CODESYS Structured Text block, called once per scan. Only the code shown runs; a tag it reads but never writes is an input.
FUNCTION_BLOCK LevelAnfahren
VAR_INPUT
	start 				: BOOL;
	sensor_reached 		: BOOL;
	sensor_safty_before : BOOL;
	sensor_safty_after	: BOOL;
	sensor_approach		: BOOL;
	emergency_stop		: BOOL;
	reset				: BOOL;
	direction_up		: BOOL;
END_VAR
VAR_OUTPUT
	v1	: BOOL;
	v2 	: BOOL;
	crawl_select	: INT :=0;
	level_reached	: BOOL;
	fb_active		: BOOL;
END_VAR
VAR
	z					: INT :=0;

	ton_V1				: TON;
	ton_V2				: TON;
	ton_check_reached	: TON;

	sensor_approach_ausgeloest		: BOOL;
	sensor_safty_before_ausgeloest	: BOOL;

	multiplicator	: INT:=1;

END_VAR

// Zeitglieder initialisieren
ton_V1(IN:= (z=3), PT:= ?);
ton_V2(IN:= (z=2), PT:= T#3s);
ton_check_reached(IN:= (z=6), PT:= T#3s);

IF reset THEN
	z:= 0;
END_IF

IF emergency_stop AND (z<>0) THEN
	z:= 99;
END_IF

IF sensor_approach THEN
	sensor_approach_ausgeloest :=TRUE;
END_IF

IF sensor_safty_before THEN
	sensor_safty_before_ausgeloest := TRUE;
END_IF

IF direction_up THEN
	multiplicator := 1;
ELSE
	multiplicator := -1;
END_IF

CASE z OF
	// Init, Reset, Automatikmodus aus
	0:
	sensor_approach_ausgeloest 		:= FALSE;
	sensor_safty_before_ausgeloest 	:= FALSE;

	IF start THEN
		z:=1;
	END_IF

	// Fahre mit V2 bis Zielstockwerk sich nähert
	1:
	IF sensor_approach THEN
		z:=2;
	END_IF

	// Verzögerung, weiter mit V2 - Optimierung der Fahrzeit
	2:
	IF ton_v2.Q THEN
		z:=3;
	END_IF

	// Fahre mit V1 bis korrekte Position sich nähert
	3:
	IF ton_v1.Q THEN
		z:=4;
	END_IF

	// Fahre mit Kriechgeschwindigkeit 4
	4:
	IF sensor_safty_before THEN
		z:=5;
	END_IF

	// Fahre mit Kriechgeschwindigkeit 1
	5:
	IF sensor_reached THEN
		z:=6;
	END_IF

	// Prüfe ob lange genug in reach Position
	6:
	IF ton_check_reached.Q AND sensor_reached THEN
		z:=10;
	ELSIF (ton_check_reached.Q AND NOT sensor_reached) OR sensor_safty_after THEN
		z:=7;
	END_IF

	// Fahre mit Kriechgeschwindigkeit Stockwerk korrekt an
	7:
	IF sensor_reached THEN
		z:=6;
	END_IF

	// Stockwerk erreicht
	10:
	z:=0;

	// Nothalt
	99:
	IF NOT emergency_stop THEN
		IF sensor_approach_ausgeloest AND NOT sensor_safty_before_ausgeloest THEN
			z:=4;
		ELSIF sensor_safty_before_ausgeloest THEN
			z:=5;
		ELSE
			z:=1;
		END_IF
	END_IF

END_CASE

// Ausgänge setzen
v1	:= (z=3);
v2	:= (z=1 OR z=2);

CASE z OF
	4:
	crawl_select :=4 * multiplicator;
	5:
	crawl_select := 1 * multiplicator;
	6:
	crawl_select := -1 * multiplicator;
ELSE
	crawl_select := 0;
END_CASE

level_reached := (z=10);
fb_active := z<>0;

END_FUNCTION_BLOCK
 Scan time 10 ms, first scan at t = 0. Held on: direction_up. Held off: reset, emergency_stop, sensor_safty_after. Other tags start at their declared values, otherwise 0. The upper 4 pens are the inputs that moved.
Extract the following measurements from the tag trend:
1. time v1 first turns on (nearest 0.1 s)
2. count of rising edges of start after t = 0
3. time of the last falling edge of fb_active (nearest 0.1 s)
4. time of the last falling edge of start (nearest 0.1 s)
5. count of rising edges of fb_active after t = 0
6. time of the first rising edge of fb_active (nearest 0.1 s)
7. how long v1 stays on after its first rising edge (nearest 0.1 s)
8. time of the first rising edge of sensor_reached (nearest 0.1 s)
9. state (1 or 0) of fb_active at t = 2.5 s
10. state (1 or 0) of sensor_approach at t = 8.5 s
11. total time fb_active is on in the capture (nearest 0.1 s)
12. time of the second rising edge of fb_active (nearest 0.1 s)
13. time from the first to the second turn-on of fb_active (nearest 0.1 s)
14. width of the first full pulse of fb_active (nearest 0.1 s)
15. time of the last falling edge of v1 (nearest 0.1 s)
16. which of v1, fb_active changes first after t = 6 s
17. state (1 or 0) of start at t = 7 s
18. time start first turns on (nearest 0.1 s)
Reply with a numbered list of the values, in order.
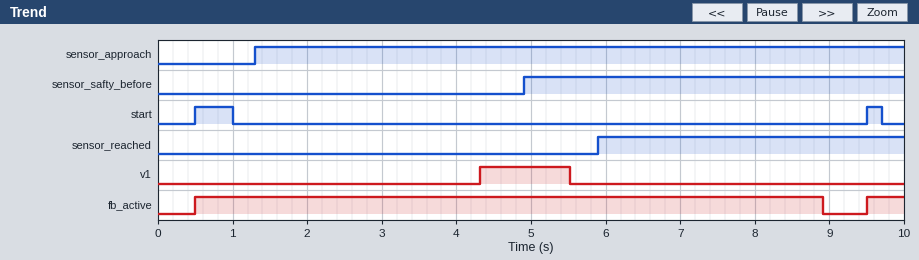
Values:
1. 4.3 s
2. 2
3. 8.9 s
4. 9.7 s
5. 2
6. 0.5 s
7. 1.2 s
8. 5.9 s
9. 1
10. 1
11. 8.9 s
12. 9.5 s
13. 9.0 s
14. 8.4 s
15. 5.5 s
16. fb_active
17. 0
18. 0.5 s
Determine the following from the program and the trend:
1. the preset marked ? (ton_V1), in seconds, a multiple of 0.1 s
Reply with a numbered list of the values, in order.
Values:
1. 1.2 s
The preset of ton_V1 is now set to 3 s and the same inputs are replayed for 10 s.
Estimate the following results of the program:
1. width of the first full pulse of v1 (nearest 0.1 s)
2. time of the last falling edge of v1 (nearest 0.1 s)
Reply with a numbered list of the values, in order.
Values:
1. 3.0 s
2. 7.3 s
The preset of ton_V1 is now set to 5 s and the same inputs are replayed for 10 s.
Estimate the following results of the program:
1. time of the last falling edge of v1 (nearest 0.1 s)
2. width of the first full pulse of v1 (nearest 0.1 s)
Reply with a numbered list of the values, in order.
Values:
1. 9.3 s
2. 5.0 s
